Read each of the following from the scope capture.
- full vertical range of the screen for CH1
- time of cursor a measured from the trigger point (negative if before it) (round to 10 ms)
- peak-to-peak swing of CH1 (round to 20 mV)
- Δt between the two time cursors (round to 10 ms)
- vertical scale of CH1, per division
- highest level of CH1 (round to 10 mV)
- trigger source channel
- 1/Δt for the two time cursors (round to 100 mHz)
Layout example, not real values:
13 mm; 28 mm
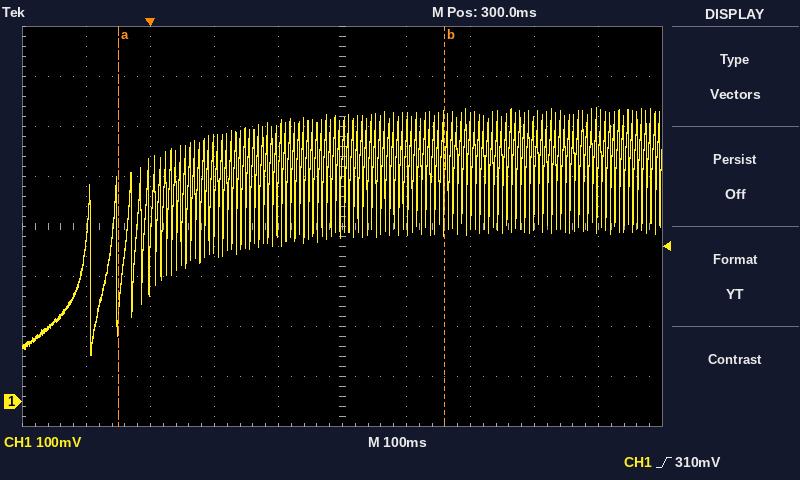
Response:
800 mV; -50 ms; 500 mV; 510 ms; 100 mV; 590 mV; CH1; 2.0 Hz
